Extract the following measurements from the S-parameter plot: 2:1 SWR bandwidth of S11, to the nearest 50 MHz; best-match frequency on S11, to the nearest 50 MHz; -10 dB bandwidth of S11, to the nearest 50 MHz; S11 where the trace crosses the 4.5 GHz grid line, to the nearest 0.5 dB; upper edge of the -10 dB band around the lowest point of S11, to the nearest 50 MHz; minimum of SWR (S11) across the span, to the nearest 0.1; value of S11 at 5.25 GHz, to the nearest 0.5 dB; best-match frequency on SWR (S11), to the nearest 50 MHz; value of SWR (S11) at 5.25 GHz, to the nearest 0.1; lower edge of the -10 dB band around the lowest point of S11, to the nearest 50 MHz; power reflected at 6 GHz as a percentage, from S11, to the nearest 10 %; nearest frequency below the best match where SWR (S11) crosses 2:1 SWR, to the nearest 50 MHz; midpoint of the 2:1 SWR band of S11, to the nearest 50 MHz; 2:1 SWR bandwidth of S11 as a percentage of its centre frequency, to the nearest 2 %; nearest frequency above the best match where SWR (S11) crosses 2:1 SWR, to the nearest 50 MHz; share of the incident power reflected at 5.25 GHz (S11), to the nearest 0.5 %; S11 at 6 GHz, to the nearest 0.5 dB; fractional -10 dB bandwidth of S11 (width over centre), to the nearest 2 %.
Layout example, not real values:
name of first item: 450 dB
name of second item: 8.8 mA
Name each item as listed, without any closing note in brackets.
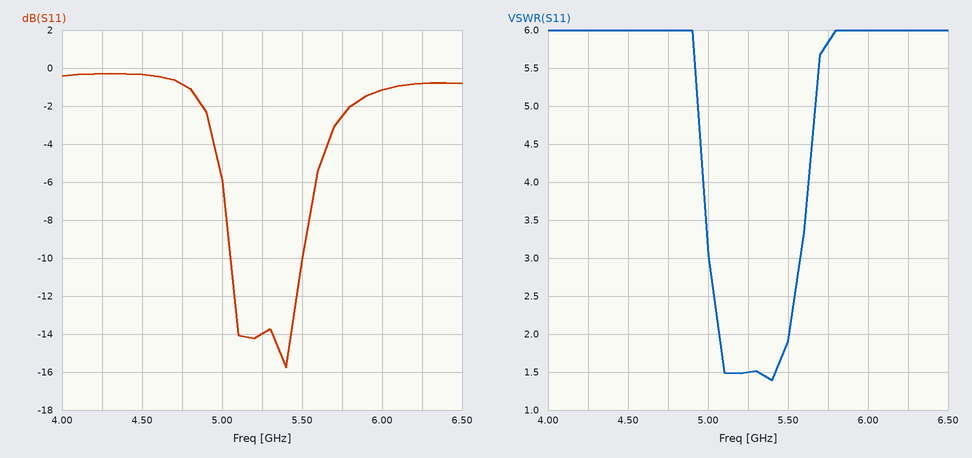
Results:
2:1 SWR bandwidth of S11, to the nearest 50 MHz: 450 MHz
best-match frequency on S11, to the nearest 50 MHz: 5.40 GHz
-10 dB bandwidth of S11, to the nearest 50 MHz: 450 MHz
S11 where the trace crosses the 4.5 GHz grid line, to the nearest 0.5 dB: -0.5 dB
upper edge of the -10 dB band around the lowest point of S11, to the nearest 50 MHz: 5.50 GHz
minimum of SWR (S11) across the span, to the nearest 0.1: 1.4
value of S11 at 5.25 GHz, to the nearest 0.5 dB: -14.0 dB
best-match frequency on SWR (S11), to the nearest 50 MHz: 5.40 GHz
value of SWR (S11) at 5.25 GHz, to the nearest 0.1: 1.5
lower edge of the -10 dB band around the lowest point of S11, to the nearest 50 MHz: 5.05 GHz
power reflected at 6 GHz as a percentage, from S11, to the nearest 10 %: 80 %
nearest frequency below the best match where SWR (S11) crosses 2:1 SWR, to the nearest 50 MHz: 5.05 GHz
midpoint of the 2:1 SWR band of S11, to the nearest 50 MHz: 5.30 GHz
2:1 SWR bandwidth of S11 as a percentage of its centre frequency, to the nearest 2 %: 8 %
nearest frequency above the best match where SWR (S11) crosses 2:1 SWR, to the nearest 50 MHz: 5.50 GHz
share of the incident power reflected at 5.25 GHz (S11), to the nearest 0.5 %: 4.0 %
S11 at 6 GHz, to the nearest 0.5 dB: -1.0 dB
fractional -10 dB bandwidth of S11 (width over centre), to the nearest 2 %: 8 %
